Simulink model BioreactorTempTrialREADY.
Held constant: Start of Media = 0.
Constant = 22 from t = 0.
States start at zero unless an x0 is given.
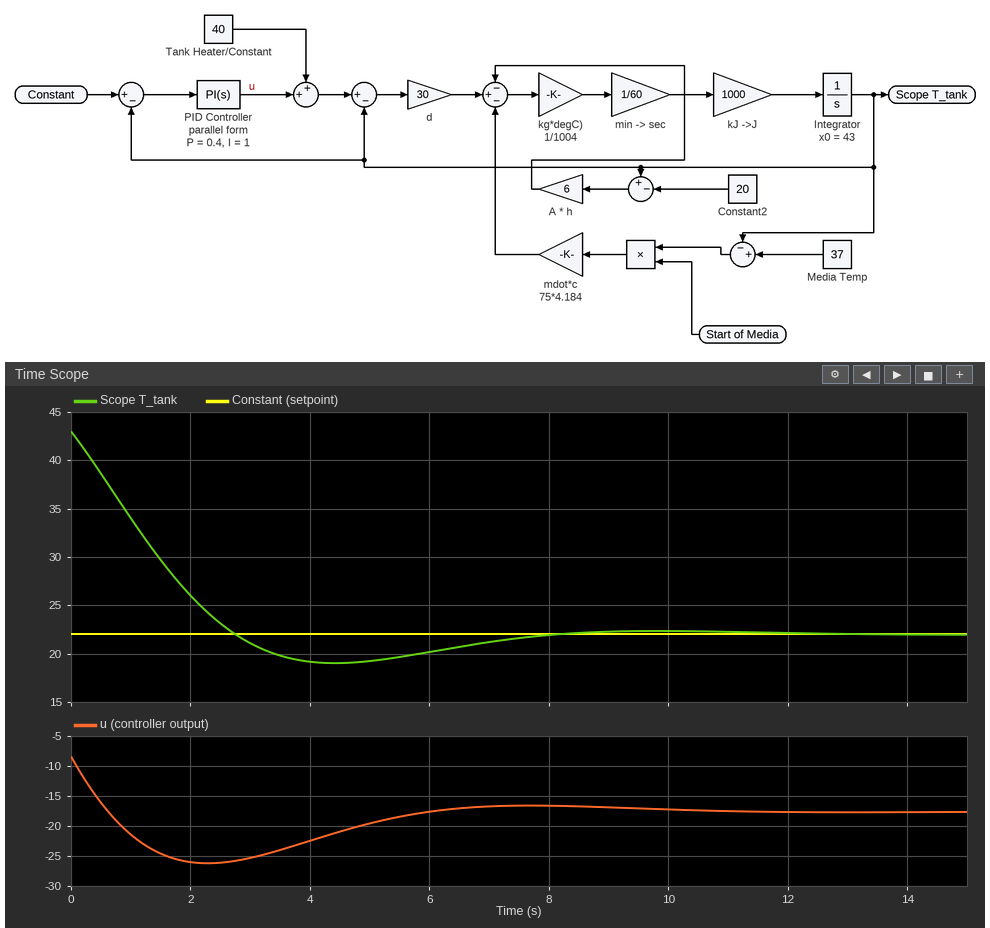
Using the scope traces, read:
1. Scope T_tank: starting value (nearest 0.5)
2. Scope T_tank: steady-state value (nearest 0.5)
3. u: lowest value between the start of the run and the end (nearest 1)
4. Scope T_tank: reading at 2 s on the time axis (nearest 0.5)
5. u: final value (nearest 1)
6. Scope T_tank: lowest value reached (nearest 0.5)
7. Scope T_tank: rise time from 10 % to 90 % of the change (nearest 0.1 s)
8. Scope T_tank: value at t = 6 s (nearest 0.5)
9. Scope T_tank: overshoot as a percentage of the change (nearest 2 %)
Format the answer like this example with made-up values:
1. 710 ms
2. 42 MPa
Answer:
1. 43.0
2. 22.0
3. -26
4. 26.0
5. -18
6. 19.0
7. 2.1 s
8. 20.0
9. 14 %
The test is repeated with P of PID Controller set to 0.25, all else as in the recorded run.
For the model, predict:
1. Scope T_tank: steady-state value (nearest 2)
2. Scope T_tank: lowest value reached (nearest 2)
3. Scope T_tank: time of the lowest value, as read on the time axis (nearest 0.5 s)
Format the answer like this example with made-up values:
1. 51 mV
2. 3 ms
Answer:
1. 22
2. 18
3. 4.5 s
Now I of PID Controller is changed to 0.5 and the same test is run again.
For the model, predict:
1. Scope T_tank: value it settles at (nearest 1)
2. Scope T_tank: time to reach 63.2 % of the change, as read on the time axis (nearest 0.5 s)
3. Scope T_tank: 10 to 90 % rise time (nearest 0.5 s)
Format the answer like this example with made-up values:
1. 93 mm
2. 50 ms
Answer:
1. 22
2. 2.0 s
3. 3.5 s
